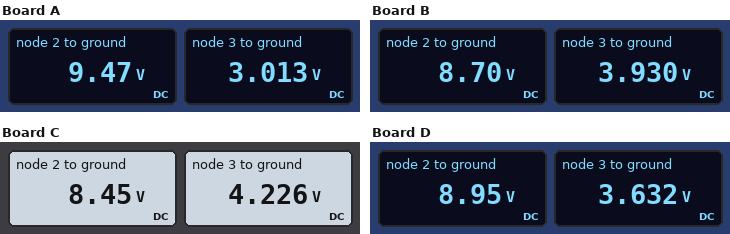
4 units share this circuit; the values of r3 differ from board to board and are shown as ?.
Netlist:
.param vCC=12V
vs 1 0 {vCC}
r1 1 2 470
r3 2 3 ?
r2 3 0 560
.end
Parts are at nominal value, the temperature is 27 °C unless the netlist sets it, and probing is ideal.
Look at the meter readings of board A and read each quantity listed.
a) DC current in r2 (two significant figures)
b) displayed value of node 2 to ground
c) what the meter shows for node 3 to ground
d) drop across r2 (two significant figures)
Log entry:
5.4 mA
9.47 V
3.013 V
3.0 V
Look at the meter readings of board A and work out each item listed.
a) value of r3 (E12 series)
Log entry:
1.2 kΩ
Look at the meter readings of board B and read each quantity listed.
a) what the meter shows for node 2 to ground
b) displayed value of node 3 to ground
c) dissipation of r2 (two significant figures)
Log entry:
8.70 V
3.930 V
28 mW
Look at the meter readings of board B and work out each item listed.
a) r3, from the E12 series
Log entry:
680 Ω
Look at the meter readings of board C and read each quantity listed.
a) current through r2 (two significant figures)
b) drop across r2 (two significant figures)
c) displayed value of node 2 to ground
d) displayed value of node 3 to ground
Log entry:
7.5 mA
4.2 V
8.45 V
4.226 V
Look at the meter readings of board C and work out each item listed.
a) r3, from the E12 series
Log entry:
560 Ω
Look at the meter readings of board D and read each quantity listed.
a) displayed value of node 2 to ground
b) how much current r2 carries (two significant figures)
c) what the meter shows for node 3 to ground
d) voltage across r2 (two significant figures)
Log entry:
8.95 V
6.5 mA
3.632 V
3.6 V
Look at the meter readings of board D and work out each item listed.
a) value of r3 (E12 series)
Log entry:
820 Ω
